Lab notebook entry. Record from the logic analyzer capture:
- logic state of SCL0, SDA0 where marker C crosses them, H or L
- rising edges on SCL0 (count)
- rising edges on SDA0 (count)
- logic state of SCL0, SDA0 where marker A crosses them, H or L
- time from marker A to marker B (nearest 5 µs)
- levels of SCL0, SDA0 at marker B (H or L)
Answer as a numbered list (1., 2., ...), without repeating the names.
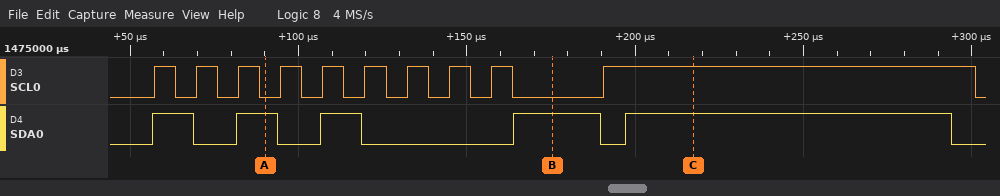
1. SCL0=H, SDA0=H
2. 10
3. 5
4. SCL0=L, SDA0=H
5. 85 µs
6. SCL0=L, SDA0=H
